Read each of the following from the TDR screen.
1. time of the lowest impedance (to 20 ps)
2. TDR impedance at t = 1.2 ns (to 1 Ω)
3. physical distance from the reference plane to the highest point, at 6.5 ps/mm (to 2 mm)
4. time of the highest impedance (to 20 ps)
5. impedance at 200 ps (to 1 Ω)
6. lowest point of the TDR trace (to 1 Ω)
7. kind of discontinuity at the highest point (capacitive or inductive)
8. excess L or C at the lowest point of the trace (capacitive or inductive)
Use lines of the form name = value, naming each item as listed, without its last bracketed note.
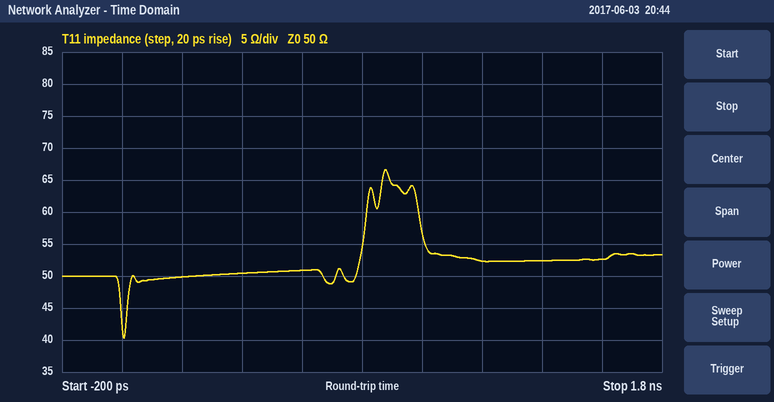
time of the lowest impedance = 0 ps
TDR impedance at t = 1.2 ns = 52 Ω
physical distance from the reference plane to the highest point, at 6.5 ps/mm = 68 mm
time of the highest impedance = 880 ps
impedance at 200 ps = 50 Ω
lowest point of the TDR trace = 40 Ω
kind of discontinuity at the highest point = inductive
excess L or C at the lowest point of the trace = capacitive
